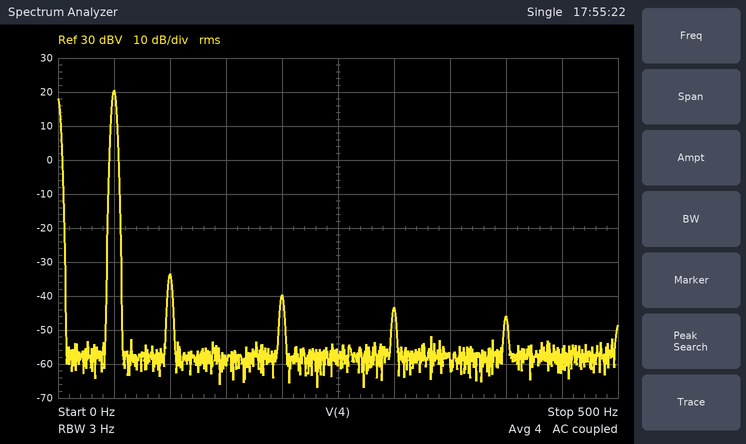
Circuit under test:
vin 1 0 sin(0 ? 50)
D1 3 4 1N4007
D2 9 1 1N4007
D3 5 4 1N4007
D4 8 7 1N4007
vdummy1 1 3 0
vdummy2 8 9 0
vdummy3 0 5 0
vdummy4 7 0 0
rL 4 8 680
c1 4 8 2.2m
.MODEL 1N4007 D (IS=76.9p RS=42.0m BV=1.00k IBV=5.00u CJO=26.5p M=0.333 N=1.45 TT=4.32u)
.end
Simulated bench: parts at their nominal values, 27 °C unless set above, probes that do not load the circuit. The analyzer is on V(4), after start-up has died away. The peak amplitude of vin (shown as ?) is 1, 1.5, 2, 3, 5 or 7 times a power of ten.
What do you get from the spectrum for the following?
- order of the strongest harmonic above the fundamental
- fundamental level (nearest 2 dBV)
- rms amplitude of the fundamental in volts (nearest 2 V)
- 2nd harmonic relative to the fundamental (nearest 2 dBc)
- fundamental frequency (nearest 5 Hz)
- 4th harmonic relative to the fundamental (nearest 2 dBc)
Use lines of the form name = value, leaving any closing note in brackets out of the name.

order of the strongest harmonic above the fundamental = 2
fundamental level = 20 dBV
rms amplitude of the fundamental in volts = 10 V
2nd harmonic relative to the fundamental = -54 dBc
fundamental frequency = 50 Hz
4th harmonic relative to the fundamental = -60 dBc
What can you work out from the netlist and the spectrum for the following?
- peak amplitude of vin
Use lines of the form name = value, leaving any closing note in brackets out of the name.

peak amplitude of vin = 30 V
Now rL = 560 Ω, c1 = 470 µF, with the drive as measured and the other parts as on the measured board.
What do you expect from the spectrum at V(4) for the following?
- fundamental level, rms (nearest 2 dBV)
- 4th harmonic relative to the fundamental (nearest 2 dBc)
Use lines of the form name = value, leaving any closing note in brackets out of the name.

fundamental level, rms = 20 dBV
4th harmonic relative to the fundamental = -46 dBc
